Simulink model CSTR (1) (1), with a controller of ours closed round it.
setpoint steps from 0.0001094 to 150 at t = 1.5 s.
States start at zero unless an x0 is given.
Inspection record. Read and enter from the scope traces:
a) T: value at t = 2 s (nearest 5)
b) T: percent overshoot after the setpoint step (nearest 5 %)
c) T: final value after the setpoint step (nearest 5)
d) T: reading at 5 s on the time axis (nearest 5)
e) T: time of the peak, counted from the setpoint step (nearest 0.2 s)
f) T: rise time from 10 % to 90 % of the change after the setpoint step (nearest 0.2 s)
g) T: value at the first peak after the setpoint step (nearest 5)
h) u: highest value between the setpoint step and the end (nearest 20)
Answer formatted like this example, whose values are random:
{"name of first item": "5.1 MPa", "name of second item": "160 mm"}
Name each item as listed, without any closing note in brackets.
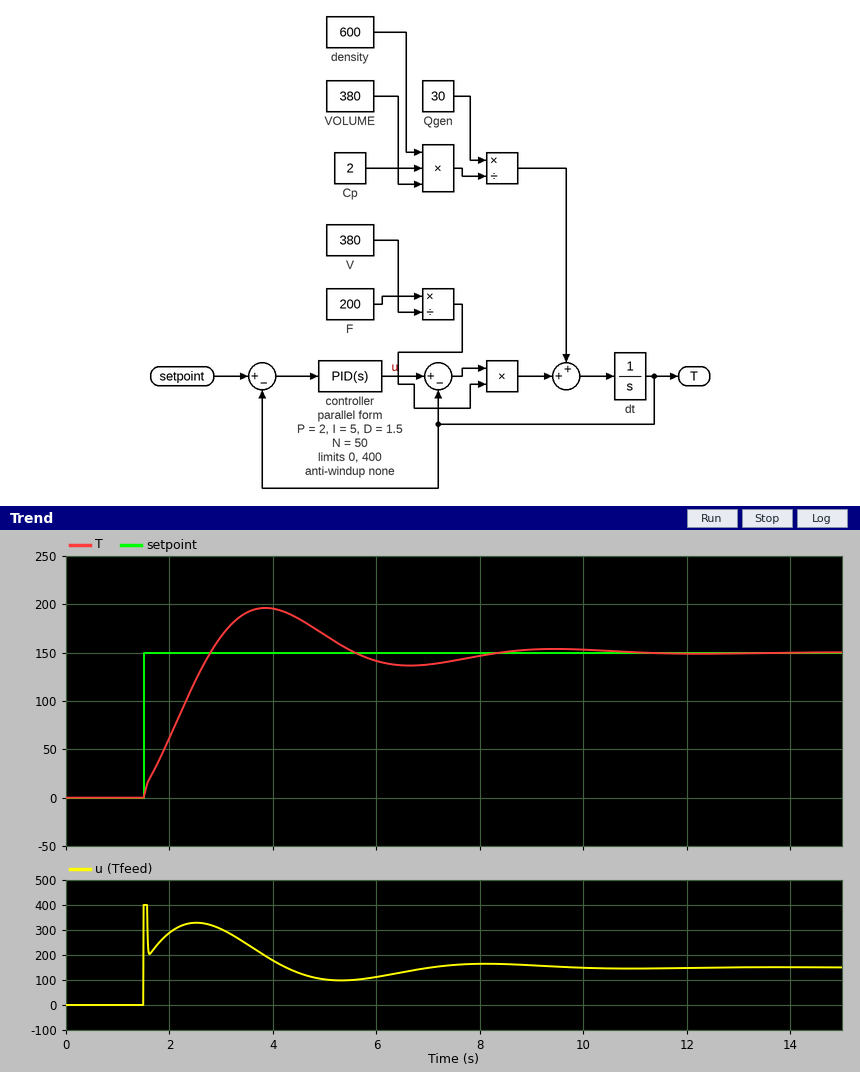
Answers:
{"T: value at t = 2 s": "60", "T: percent overshoot after the setpoint step": "30 %", "T: final value after the setpoint step": "150", "T: reading at 5 s on the time axis": "170", "T: time of the peak, counted from the setpoint step": "2.4 s", "T: rise time from 10 % to 90 % of the change after the setpoint step": "1.0 s", "T: value at the first peak after the setpoint step": "195", "u: highest value between the setpoint step and the end": "400"}
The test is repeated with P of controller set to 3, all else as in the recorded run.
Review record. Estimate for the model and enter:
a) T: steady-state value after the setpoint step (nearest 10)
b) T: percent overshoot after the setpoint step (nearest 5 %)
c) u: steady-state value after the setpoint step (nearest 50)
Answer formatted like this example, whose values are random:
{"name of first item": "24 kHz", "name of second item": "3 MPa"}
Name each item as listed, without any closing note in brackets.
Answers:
{"T: steady-state value after the setpoint step": "150", "T: percent overshoot after the setpoint step": "25 %", "u: steady-state value after the setpoint step": "150"}
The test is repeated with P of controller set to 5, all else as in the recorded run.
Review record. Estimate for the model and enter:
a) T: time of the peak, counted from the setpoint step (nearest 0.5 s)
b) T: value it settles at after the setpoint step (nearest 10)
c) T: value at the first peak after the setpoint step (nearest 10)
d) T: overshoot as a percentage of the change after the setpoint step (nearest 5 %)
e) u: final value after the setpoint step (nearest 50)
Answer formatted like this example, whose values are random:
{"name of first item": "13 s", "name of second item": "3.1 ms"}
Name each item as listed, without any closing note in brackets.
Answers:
{"T: time of the peak, counted from the setpoint step": "2.0 s", "T: value it settles at after the setpoint step": "150", "T: value at the first peak after the setpoint step": "170", "T: overshoot as a percentage of the change after the setpoint step": "15 %", "u: final value after the setpoint step": "150"}
